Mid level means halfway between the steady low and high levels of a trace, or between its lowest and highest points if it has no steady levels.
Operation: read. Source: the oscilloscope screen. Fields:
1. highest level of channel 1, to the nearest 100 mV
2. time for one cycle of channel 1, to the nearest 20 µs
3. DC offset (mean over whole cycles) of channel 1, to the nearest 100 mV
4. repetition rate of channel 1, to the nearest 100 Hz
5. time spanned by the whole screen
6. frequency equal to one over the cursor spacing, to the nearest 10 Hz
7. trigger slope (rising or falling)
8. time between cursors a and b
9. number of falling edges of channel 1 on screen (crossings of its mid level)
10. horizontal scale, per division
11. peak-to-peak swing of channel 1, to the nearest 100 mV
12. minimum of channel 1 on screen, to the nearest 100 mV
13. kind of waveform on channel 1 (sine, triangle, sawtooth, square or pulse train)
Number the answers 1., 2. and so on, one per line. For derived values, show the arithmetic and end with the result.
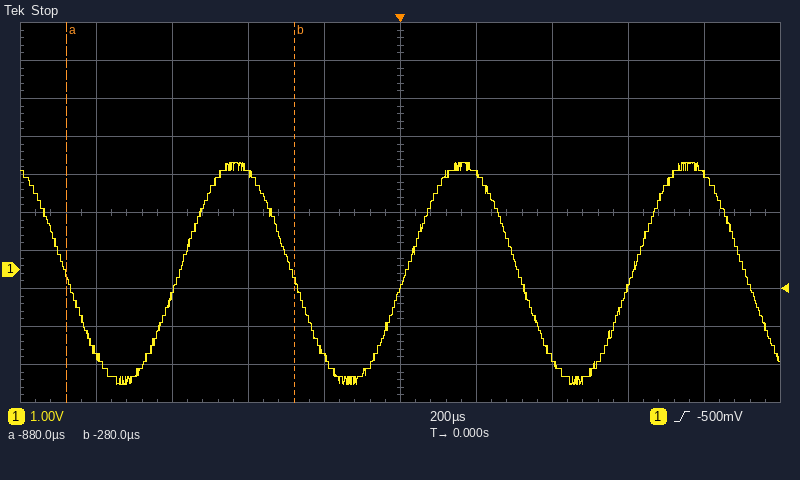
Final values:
1. 2.8 V
2. 600 µs
3. (2.8 V + (-3.0 V)) / 2 ≈ -100 mV
4. 1 / 600 µs ≈ 1.7 kHz
5. 2 ms
6. 1 / 600 µs ≈ 1.67 kHz
7. rising
8. -280 µs − (-880 µs) = 600 µs
9. 4
10. 200 µs
11. 2.8 V − (-3.0 V) = 5.8 V
12. -3.0 V
13. sine
